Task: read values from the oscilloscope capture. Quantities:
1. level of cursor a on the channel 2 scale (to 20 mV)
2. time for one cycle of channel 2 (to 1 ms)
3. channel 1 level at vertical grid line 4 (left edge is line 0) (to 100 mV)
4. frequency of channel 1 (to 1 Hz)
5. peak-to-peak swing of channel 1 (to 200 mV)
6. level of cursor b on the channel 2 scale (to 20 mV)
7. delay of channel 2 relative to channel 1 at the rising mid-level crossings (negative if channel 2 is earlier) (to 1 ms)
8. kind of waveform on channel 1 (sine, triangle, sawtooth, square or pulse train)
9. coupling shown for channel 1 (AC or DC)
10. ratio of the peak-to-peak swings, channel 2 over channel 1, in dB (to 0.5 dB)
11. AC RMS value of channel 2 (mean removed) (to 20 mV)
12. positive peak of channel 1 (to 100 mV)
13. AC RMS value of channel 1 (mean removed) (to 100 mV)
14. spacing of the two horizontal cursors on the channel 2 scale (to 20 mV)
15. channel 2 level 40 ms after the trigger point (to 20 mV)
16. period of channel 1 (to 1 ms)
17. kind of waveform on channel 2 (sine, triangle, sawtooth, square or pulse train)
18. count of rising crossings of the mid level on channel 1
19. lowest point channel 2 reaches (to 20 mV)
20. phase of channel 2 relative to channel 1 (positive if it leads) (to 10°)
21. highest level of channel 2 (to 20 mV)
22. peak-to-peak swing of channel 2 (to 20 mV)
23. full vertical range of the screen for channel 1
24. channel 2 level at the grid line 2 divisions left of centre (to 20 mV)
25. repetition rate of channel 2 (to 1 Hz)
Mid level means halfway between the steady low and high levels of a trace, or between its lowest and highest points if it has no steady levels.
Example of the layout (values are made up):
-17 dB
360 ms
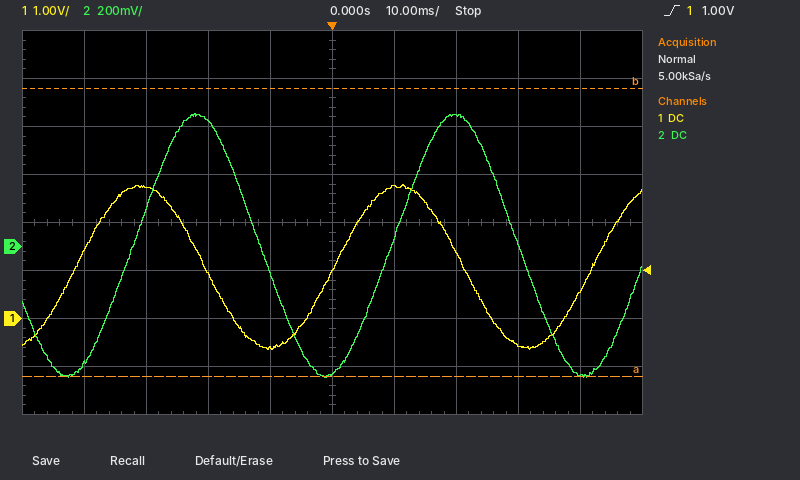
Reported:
-540 mV
42 ms
-600 mV
24 Hz
3.4 V
660 mV
+9 ms
sine
DC
-10.0 dB
380 mV
2.8 V
1.2 V
1.20 V
-540 mV
42 ms
sine
3
-540 mV
-80°
560 mV
1.10 V
8 V
520 mV
24 Hz
